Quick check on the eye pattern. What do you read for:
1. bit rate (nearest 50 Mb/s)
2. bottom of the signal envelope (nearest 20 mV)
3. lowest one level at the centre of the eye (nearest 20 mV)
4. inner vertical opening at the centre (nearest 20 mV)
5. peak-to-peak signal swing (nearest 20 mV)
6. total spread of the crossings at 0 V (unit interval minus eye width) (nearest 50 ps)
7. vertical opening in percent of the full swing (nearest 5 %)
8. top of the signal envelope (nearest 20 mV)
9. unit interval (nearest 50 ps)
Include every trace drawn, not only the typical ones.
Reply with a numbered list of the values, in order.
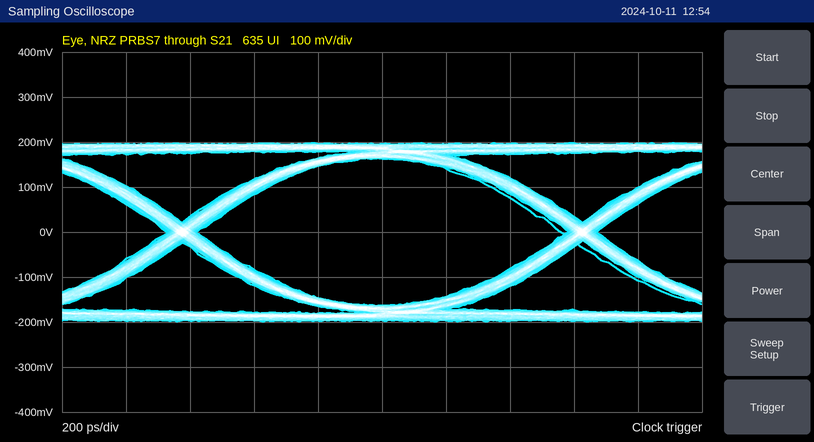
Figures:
1. 800 Mb/s
2. -200 mV
3. 160 mV
4. 320 mV
5. 400 mV
6. 100 ps
7. 80 %
8. 200 mV
9. 1.25 ns
